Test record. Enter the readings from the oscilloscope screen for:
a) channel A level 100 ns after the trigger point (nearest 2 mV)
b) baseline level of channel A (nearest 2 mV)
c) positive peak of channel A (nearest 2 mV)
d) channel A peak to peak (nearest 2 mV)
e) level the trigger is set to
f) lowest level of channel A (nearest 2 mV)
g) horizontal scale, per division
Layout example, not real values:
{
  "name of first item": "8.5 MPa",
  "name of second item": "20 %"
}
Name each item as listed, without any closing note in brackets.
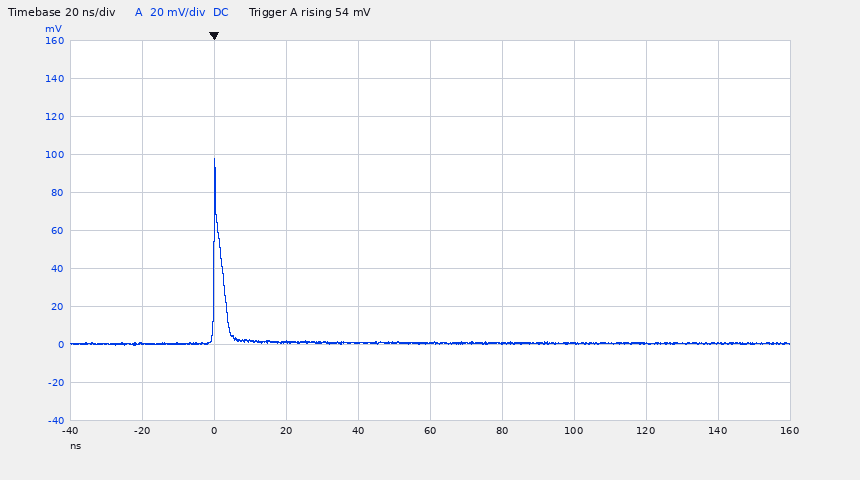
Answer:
{
  "channel A level 100 ns after the trigger point": "0 mV",
  "baseline level of channel A": "0 mV",
  "positive peak of channel A": "98 mV",
  "channel A peak to peak": "98 mV",
  "level the trigger is set to": "54 mV",
  "lowest level of channel A": "0 mV",
  "horizontal scale, per division": "20 ns"
}
